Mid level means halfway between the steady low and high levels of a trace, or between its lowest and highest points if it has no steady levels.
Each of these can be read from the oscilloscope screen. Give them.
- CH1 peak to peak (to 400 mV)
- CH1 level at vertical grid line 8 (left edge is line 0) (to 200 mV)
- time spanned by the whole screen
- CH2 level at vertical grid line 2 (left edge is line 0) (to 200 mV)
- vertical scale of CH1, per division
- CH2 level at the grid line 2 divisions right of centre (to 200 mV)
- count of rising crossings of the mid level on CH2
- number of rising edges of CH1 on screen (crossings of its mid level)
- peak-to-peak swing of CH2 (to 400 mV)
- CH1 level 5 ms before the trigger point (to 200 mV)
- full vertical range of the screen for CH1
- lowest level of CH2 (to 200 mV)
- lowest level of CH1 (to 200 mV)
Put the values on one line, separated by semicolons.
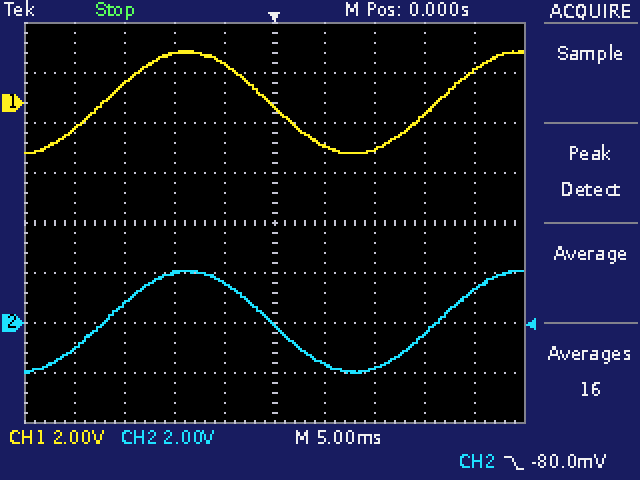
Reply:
4.0 V; -400 mV; 50 ms; 800 mV; 2 V; -1.8 V; 2; 2; 4.0 V; 1.6 V; 16 V; -2.0 V; -2.0 V
